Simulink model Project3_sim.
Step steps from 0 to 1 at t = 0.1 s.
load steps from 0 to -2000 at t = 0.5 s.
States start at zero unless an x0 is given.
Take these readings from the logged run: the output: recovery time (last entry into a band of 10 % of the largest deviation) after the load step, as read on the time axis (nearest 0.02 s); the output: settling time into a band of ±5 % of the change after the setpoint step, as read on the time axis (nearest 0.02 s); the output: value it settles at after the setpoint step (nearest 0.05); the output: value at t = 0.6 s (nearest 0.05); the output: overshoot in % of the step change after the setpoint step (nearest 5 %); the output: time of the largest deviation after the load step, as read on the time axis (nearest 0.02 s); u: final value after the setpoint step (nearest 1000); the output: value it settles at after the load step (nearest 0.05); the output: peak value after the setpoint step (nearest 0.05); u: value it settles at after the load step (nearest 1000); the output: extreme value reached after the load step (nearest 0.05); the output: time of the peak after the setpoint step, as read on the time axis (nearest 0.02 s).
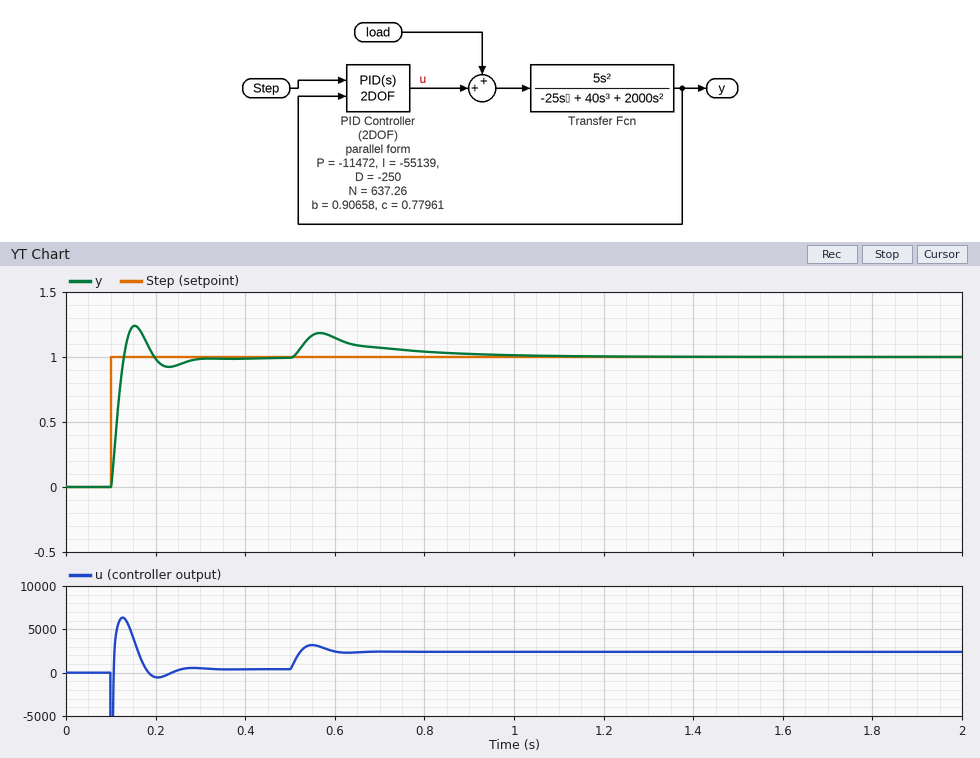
0.94 s
0.26 s
1.00
1.15
25 %
0.56 s
0
1.00
1.25
2000
1.20
0.16 s
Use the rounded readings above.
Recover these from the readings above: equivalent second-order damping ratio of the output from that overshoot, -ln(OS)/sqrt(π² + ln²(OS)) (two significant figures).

0.40
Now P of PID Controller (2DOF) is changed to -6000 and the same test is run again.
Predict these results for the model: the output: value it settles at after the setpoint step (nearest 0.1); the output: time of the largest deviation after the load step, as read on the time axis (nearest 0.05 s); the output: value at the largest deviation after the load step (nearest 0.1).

1.0
0.60 s
1.3
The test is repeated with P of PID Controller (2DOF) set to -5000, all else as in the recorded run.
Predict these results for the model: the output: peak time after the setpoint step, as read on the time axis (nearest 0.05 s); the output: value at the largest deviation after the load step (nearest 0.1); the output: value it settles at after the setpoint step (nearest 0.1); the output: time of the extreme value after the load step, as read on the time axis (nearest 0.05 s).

0.20 s
1.3
1.0
0.60 s
